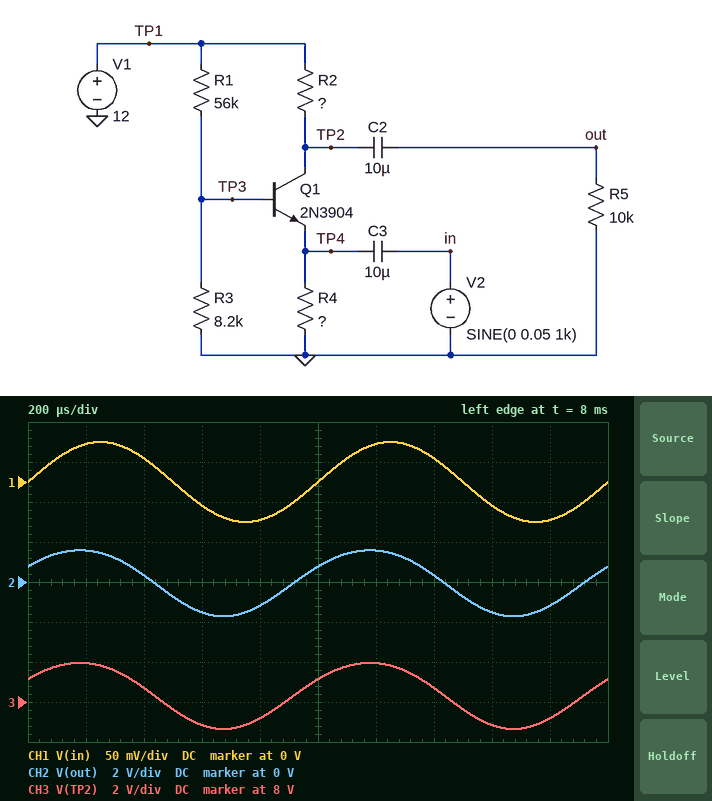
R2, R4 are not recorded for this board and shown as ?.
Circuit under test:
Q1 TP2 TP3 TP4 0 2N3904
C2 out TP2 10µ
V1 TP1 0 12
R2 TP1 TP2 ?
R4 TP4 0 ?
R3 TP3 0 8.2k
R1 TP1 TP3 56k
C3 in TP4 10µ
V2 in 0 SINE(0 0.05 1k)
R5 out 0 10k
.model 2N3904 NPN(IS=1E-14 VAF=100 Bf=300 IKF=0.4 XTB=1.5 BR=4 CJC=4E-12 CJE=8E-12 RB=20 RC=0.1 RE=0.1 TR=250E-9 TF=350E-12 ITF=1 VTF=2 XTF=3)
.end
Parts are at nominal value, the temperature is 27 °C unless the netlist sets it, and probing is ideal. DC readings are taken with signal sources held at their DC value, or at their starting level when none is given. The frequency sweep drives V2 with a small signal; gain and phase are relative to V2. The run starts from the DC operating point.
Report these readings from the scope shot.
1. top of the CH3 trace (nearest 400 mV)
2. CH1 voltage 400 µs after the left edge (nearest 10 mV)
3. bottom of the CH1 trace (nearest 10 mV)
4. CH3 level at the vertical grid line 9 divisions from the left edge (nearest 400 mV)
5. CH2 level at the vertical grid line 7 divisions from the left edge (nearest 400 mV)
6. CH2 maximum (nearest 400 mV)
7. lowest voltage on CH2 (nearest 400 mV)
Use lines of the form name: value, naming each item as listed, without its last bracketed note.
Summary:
top of the CH3 trace: 10.0 V
CH1 voltage 400 µs after the left edge: 30 mV
bottom of the CH1 trace: -50 mV
CH3 level at the vertical grid line 9 divisions from the left edge: 7.2 V
CH2 level at the vertical grid line 7 divisions from the left edge: 400 mV
CH2 maximum: 1.6 V
lowest voltage on CH2: -1.6 V
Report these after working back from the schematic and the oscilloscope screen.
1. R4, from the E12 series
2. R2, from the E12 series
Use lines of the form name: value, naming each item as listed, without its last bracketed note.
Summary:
R4, from the E12 series: 330 Ω
R2, from the E12 series: 1.5 kΩ
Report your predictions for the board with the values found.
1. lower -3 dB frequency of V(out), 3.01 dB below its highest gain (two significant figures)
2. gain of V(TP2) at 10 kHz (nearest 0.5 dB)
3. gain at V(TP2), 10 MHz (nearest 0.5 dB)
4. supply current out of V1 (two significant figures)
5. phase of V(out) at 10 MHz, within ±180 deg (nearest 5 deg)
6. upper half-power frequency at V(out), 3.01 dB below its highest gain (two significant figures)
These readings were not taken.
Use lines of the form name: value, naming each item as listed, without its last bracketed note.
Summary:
lower -3 dB frequency of V(out), 3.01 dB below its highest gain: 510 Hz
gain of V(TP2) at 10 kHz: 31.5 dB
gain at V(TP2), 10 MHz: 2.0 dB
supply current out of V1: 2.6 mA
phase of V(out) at 10 MHz, within ±180 deg: -50 deg
upper half-power frequency at V(out), 3.01 dB below its highest gain: 260 kHz
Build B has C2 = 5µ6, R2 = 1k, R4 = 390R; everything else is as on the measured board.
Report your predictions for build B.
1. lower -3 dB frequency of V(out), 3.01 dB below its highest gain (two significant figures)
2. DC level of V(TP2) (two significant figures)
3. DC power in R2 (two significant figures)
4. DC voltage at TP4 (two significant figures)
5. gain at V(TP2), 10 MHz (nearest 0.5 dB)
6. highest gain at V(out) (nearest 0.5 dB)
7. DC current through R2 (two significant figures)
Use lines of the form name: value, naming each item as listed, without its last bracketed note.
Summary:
lower -3 dB frequency of V(out), 3.01 dB below its highest gain: 490 Hz
DC level of V(TP2): 9.9 V
DC power in R2: 4.3 mW
DC voltage at TP4: 810 mV
gain at V(TP2), 10 MHz: 1.5 dB
highest gain at V(out): 28.0 dB
DC current through R2: 2.1 mA
